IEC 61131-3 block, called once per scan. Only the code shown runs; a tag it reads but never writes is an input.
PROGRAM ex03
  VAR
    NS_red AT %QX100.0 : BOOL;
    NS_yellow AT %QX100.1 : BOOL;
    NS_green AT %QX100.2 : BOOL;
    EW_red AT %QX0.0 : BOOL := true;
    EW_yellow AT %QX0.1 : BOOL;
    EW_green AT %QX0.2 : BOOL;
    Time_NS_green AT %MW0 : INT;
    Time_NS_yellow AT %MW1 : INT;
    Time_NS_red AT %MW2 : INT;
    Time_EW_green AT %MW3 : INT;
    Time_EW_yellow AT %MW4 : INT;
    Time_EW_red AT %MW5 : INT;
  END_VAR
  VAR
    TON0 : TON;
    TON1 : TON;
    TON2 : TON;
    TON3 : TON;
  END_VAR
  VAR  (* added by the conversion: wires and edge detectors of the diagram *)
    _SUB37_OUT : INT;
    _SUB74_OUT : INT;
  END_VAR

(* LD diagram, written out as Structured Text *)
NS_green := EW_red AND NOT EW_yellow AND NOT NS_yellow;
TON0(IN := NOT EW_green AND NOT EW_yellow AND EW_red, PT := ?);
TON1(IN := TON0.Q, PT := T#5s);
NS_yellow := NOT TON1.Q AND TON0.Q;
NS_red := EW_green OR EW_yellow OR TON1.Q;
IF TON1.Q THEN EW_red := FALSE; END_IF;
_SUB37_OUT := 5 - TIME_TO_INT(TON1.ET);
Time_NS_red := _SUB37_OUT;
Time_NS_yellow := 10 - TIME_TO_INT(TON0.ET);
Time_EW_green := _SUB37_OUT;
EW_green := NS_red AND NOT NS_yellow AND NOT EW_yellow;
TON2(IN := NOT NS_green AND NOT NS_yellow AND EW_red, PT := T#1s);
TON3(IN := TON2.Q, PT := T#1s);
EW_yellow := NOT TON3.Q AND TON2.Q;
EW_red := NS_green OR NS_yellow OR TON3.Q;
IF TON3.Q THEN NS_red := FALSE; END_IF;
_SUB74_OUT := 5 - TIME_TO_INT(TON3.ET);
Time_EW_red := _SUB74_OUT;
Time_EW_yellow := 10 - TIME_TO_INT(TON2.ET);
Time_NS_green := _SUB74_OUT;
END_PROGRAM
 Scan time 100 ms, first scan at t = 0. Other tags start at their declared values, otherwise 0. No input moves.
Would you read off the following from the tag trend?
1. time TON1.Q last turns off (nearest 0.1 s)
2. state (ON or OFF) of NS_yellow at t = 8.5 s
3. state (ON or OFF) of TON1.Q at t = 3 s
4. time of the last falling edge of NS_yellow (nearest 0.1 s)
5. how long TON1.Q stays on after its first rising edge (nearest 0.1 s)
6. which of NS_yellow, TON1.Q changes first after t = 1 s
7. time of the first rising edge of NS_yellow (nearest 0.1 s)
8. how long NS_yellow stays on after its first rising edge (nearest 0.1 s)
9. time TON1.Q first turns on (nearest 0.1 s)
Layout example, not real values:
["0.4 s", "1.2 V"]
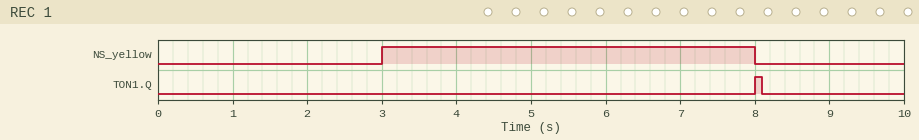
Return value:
["8.1 s", "OFF", "OFF", "8.0 s", "0.1 s", "NS_yellow", "3.0 s", "5.0 s", "8.0 s"]
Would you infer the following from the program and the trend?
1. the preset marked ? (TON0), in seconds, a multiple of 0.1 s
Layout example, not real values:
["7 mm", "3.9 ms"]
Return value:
["3.0 s"]
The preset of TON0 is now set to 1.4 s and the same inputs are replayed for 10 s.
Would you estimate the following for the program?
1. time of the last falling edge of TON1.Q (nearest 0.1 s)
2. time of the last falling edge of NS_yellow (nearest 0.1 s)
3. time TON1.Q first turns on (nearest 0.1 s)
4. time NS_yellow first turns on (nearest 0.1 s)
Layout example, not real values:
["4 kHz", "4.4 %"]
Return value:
["6.5 s", "6.4 s", "6.4 s", "1.4 s"]
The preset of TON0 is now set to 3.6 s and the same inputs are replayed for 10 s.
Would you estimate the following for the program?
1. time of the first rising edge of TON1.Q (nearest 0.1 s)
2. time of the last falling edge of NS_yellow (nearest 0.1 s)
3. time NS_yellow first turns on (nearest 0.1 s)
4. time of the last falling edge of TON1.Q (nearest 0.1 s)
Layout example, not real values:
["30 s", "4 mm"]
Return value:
["8.6 s", "8.6 s", "3.6 s", "8.7 s"]
